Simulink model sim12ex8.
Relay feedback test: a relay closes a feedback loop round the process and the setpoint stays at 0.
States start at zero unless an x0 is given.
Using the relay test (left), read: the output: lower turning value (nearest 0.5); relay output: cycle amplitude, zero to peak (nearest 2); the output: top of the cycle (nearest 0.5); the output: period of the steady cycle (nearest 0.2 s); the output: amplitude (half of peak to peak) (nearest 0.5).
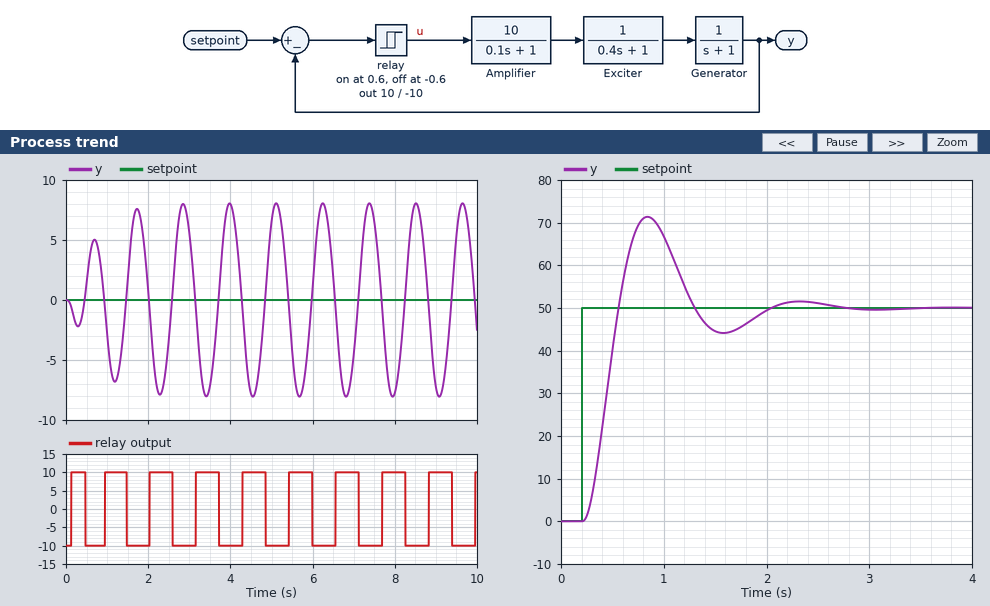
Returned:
-8.0
10
8.0
1.2 s
8.0
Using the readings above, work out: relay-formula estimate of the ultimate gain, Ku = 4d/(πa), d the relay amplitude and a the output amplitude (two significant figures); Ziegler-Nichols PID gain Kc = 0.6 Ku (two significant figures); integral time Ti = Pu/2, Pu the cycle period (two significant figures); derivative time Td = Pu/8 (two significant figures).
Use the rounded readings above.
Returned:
1.6
0.96
0.60 s
0.15 s
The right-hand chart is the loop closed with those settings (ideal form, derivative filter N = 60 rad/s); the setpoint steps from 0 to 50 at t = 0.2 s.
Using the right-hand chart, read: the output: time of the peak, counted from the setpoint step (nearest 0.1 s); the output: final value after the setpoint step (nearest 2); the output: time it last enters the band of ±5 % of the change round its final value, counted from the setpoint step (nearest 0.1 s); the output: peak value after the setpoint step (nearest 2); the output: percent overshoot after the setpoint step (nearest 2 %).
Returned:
0.6 s
50
1.7 s
72
42 %
